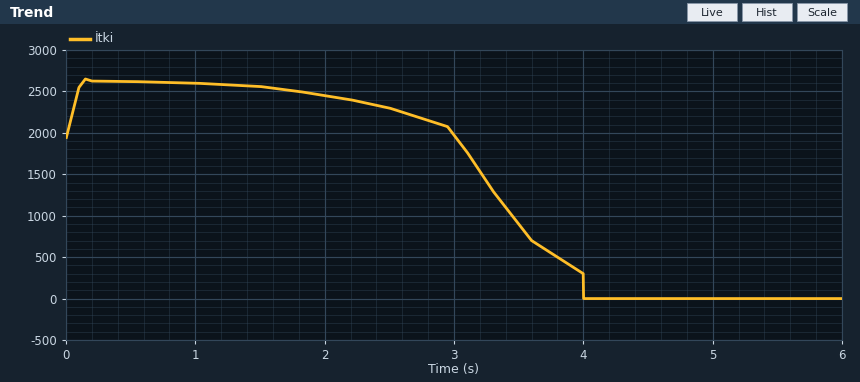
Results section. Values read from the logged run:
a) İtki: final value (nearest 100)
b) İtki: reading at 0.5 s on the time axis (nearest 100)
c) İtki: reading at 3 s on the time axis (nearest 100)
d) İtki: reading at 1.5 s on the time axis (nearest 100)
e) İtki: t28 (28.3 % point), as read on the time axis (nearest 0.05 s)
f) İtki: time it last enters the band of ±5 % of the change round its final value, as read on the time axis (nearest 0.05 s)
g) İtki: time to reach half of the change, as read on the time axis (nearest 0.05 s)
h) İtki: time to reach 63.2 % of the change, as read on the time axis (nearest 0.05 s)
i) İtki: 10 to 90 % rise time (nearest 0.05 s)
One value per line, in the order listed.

0
2600
2000
2600
3.25 s
4.00 s
3.45 s
3.60 s
0.90 s
